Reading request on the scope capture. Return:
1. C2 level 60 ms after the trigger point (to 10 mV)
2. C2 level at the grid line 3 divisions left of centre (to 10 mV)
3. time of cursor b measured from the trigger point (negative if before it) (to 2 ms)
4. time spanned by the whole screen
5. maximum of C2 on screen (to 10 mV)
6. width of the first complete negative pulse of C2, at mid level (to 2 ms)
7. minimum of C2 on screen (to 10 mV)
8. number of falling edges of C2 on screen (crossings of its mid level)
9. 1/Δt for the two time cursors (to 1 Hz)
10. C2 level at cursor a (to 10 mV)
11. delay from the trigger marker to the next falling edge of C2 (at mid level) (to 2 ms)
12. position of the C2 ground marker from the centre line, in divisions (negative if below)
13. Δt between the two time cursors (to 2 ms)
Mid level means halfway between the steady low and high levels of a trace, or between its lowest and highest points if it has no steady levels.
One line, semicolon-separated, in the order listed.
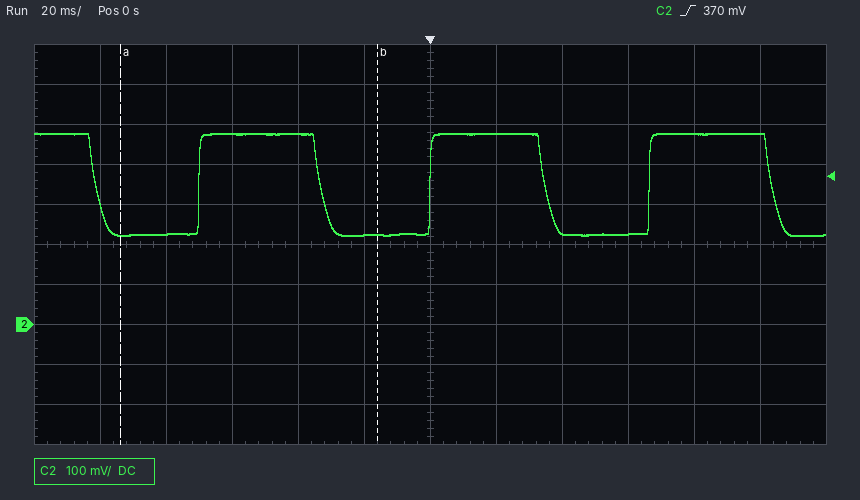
230 mV; 480 mV; -16 ms; 240 ms; 480 mV; 32 ms; 220 mV; 4; 13 Hz; 220 mV; 34 ms; -2.0 div; 78 ms
